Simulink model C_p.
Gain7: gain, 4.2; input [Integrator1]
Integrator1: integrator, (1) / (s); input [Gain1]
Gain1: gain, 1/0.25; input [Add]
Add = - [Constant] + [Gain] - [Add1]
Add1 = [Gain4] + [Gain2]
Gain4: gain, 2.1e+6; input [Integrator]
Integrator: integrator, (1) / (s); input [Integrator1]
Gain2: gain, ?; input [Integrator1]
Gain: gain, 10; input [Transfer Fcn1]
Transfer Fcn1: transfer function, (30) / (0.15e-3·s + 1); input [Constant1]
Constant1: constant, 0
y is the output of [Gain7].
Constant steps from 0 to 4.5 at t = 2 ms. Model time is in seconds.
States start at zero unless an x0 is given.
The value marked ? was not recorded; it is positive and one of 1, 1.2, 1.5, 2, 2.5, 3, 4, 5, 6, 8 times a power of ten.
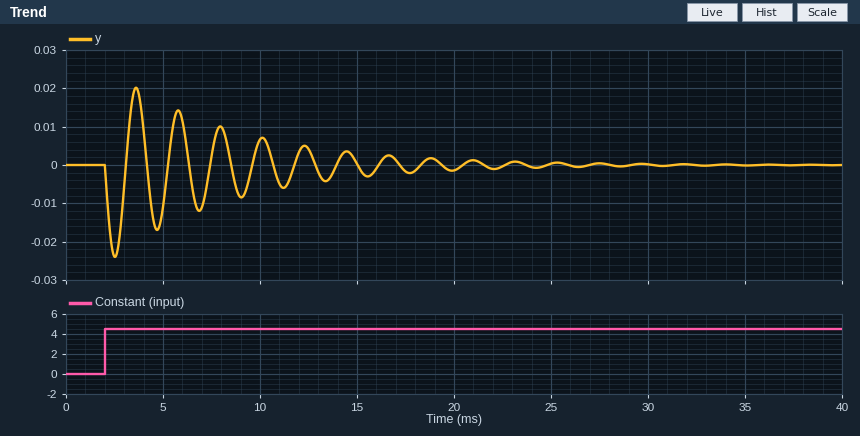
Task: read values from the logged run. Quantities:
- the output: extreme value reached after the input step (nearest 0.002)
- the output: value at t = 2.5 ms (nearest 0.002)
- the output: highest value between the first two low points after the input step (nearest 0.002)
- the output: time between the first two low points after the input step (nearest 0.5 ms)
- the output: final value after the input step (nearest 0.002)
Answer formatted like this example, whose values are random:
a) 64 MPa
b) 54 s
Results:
a) -0.024
b) -0.024
c) 0.020
d) 2.0 ms
e) 0.000
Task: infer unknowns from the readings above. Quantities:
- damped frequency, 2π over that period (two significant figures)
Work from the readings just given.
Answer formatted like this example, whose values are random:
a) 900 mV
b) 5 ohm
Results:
a) 3.1 rad/ms
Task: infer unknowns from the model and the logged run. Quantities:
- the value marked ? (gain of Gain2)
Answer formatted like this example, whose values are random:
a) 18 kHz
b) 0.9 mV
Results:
a) 80
